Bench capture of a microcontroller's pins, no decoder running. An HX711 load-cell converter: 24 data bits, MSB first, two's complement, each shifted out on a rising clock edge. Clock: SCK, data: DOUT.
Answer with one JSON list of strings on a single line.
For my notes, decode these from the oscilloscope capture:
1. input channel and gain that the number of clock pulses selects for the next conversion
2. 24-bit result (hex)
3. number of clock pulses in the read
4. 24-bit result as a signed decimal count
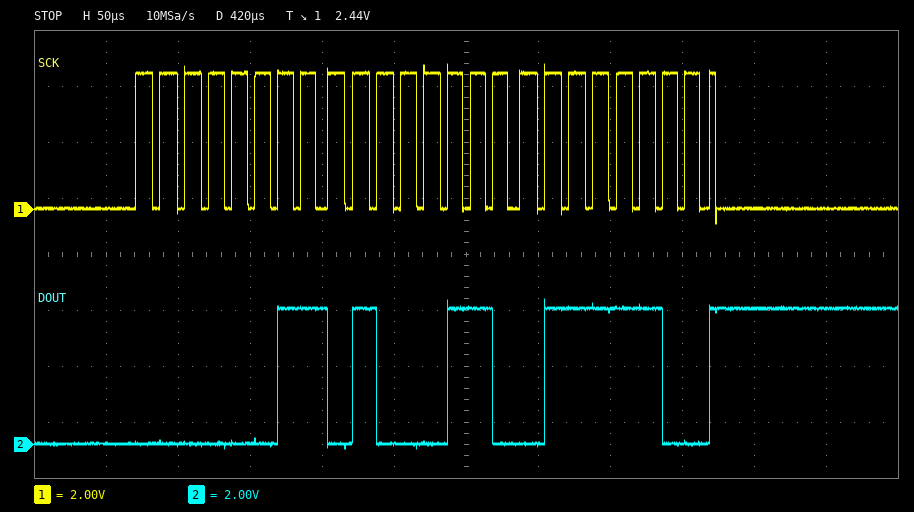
["channel A, gain 128", "0x03467C", "25", "214652"]
